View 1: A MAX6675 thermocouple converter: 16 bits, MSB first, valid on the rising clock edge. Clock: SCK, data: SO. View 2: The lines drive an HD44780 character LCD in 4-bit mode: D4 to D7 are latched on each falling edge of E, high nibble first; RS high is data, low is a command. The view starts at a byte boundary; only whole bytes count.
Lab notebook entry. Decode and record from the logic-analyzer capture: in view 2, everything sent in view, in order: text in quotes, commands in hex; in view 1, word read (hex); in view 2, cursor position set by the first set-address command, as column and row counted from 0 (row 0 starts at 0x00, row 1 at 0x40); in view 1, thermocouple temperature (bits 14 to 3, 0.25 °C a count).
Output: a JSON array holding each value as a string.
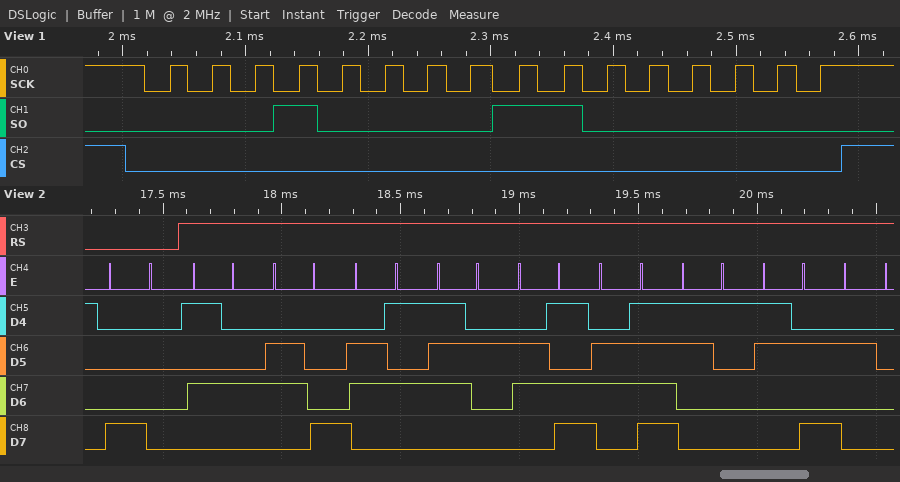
["0x80 \"Thermo1: \"", "0x10C0", "column 0, row 0", "134.00 °C"]
